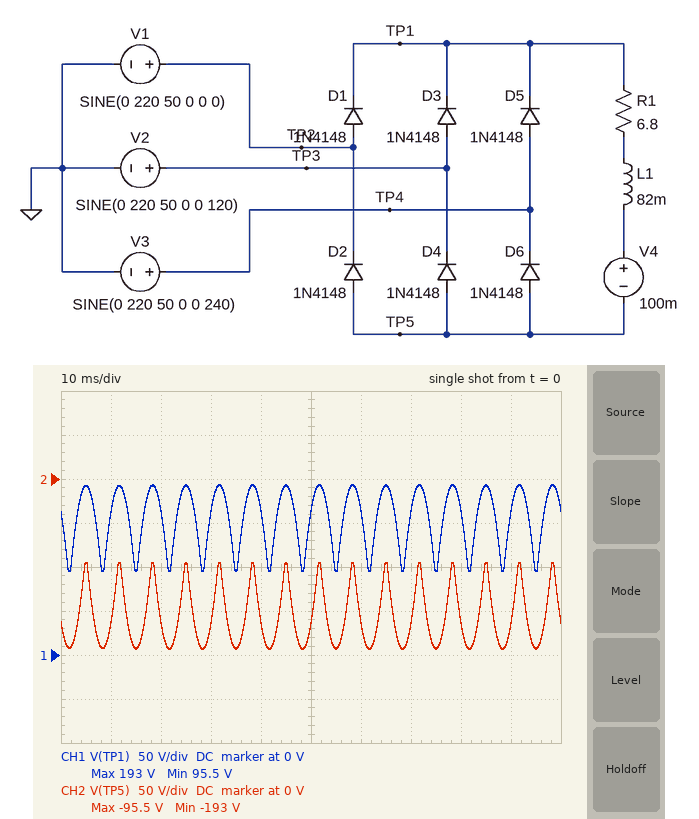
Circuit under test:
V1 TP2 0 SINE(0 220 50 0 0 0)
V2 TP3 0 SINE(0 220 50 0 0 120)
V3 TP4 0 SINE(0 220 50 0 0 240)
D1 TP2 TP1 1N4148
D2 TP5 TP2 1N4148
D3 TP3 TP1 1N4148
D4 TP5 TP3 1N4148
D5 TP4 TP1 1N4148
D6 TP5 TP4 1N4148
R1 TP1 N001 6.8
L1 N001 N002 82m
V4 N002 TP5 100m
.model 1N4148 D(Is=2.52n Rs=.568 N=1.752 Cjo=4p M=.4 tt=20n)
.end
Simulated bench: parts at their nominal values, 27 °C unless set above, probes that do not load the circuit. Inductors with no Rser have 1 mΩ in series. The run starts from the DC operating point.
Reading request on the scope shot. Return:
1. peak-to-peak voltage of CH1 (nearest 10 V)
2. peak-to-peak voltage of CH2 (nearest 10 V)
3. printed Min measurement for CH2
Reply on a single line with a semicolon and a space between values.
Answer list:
100 V; 100 V; -193 V
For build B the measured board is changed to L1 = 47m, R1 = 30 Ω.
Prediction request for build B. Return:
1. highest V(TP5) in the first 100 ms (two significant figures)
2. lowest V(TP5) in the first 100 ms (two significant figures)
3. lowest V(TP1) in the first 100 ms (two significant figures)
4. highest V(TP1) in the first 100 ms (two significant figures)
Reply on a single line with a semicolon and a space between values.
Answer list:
-110 V; -210 V; 110 V; 210 V
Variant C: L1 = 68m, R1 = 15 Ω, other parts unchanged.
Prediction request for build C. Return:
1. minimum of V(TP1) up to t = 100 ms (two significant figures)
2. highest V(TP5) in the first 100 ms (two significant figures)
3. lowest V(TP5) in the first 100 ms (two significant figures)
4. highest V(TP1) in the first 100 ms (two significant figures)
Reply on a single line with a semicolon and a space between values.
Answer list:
100 V; -100 V; -210 V; 210 V
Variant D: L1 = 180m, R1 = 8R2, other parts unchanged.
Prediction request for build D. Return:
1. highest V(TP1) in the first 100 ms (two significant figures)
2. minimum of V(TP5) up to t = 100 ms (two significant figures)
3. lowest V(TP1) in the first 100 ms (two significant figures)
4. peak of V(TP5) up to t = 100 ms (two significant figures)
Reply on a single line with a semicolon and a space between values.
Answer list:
200 V; -200 V; 97 V; -97 V
